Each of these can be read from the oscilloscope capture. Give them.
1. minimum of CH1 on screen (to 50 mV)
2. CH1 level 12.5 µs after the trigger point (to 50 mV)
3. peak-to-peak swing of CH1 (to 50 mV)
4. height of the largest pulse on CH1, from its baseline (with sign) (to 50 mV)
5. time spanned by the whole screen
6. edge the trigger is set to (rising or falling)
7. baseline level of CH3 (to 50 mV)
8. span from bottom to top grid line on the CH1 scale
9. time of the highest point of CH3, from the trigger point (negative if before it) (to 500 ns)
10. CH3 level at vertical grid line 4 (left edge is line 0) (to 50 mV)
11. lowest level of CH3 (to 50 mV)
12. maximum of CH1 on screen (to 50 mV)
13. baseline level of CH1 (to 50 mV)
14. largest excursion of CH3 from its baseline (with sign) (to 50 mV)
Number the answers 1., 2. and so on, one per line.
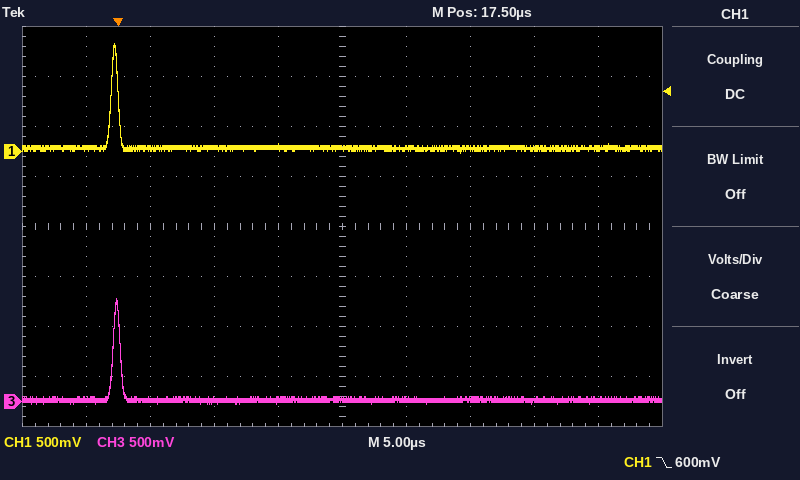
1. 0 mV
2. 50 mV
3. 1.10 V
4. +1.05 V
5. 50 µs
6. falling
7. 0 mV
8. 4 V
9. 0.0 µs
10. 0 mV
11. -50 mV
12. 1.10 V
13. 50 mV
14. +1.00 V
